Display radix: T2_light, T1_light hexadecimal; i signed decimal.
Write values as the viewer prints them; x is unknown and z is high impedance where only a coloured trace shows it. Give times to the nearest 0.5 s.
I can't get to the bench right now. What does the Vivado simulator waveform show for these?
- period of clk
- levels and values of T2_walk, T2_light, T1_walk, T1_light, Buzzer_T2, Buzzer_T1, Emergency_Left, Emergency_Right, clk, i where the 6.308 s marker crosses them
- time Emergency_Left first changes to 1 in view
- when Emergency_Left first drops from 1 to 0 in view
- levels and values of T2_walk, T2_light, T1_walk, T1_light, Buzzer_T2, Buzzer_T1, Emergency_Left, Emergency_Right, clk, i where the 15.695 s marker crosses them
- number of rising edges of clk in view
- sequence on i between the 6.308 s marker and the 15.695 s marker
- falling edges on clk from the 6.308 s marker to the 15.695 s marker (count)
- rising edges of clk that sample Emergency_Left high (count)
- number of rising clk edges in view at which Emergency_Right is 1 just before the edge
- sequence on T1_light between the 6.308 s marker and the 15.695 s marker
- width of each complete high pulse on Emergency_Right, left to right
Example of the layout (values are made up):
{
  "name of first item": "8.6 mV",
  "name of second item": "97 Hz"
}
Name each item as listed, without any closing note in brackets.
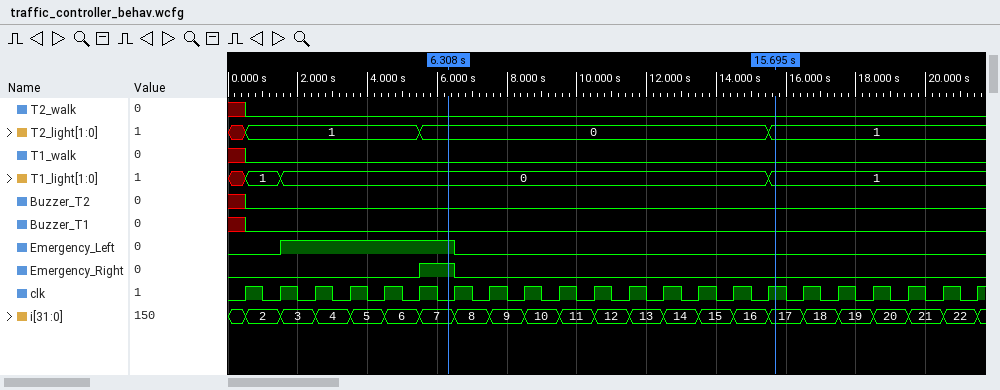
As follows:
{
  "period of clk": "1 s",
  "levels and values of T2_walk, T2_light, T1_walk, T1_light, Buzzer_T2, Buzzer_T1, Emergency_Left, Emergency_Right, clk, i where the 6.308 s marker crosses them": "T2_walk=0, T2_light=0, T1_walk=0, T1_light=0, Buzzer_T2=0, Buzzer_T1=0, Emergency_Left=1, Emergency_Right=1, clk=0, i=7",
  "time Emergency_Left first changes to 1 in view": "1.5 s",
  "when Emergency_Left first drops from 1 to 0 in view": "6.5 s",
  "levels and values of T2_walk, T2_light, T1_walk, T1_light, Buzzer_T2, Buzzer_T1, Emergency_Left, Emergency_Right, clk, i where the 15.695 s marker crosses them": "T2_walk=0, T2_light=1, T1_walk=0, T1_light=1, Buzzer_T2=0, Buzzer_T1=0, Emergency_Left=0, Emergency_Right=0, clk=1, i=17",
  "number of rising edges of clk in view": "22",
  "sequence on i between the 6.308 s marker and the 15.695 s marker": "7, 8, 9, 10, 11, 12, 13, 14, 15, 16, 17",
  "falling edges on clk from the 6.308 s marker to the 15.695 s marker": "9",
  "rising edges of clk that sample Emergency_Left high": "5",
  "number of rising clk edges in view at which Emergency_Right is 1 just before the edge": "1",
  "sequence on T1_light between the 6.308 s marker and the 15.695 s marker": "0, 1",
  "width of each complete high pulse on Emergency_Right, left to right": "1 s"
}
